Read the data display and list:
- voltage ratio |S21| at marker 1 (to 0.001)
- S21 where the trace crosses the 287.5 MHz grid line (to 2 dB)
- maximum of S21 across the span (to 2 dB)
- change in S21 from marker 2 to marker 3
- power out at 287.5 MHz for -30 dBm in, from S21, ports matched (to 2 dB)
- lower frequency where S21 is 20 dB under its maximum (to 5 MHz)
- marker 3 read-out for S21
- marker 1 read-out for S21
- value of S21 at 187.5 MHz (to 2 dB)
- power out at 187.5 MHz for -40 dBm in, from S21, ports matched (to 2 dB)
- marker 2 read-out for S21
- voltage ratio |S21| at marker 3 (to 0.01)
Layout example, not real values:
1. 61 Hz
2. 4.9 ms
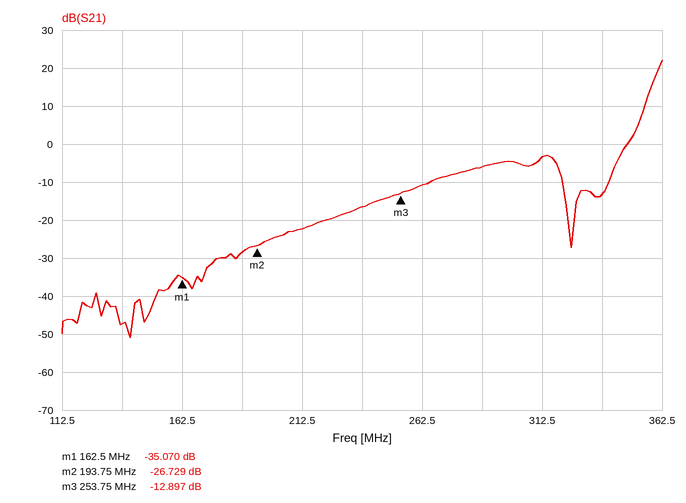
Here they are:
1. 0.018
2. -6 dB
3. 22 dB
4. 13.832 dB
5. -36 dBm
6. 350 MHz
7. -12.897 dB
8. -35.070 dB
9. -28 dB
10. -68 dBm
11. -26.729 dB
12. 0.23
